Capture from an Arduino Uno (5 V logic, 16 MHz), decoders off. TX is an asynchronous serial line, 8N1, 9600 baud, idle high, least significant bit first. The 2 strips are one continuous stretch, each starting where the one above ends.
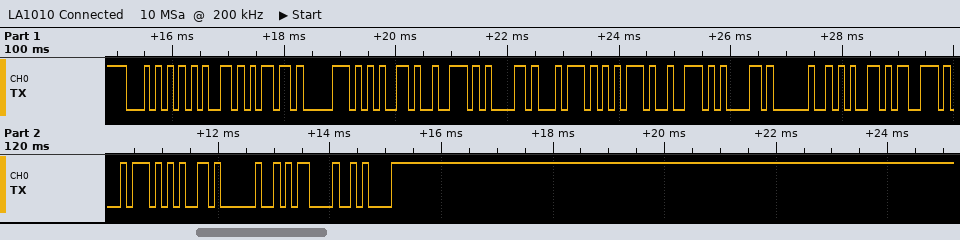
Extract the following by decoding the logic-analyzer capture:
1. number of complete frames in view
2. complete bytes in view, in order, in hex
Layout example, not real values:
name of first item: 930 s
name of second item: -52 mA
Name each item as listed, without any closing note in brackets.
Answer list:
number of complete frames in view: 19
complete bytes in view, in order, in hex: 54 65 6D 70 65 72 61 74 75 72 61 20 65 73 74 65 20 0D 0A
